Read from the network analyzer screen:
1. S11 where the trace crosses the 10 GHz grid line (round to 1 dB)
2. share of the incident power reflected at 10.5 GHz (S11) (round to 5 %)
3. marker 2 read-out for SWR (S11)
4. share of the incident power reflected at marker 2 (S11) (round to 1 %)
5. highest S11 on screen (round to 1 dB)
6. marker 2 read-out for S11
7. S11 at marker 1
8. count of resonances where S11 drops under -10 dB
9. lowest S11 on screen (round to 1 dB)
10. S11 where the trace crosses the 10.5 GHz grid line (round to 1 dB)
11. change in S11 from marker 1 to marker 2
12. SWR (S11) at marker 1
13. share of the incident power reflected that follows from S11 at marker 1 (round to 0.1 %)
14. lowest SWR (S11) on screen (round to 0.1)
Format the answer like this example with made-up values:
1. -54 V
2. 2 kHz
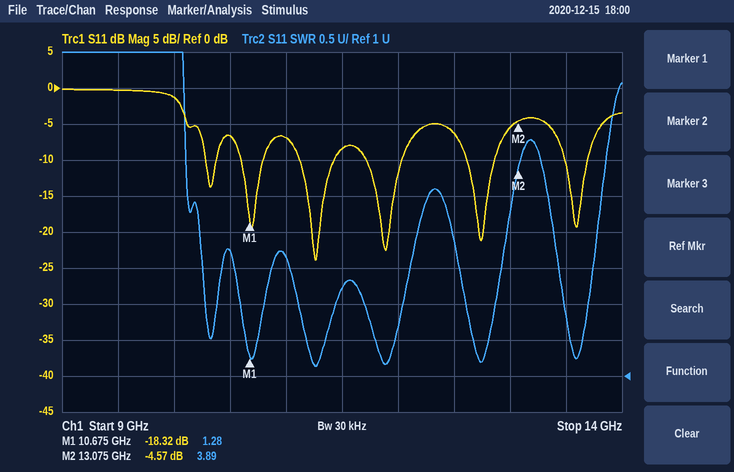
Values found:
1. -1 dB
2. 20 %
3. 3.89
4. 35 %
5. 0 dB
6. -4.57 dB
7. -18.32 dB
8. 6
9. -24 dB
10. -7 dB
11. 13.75 dB
12. 1.28
13. 1.5 %
14. 1.1
